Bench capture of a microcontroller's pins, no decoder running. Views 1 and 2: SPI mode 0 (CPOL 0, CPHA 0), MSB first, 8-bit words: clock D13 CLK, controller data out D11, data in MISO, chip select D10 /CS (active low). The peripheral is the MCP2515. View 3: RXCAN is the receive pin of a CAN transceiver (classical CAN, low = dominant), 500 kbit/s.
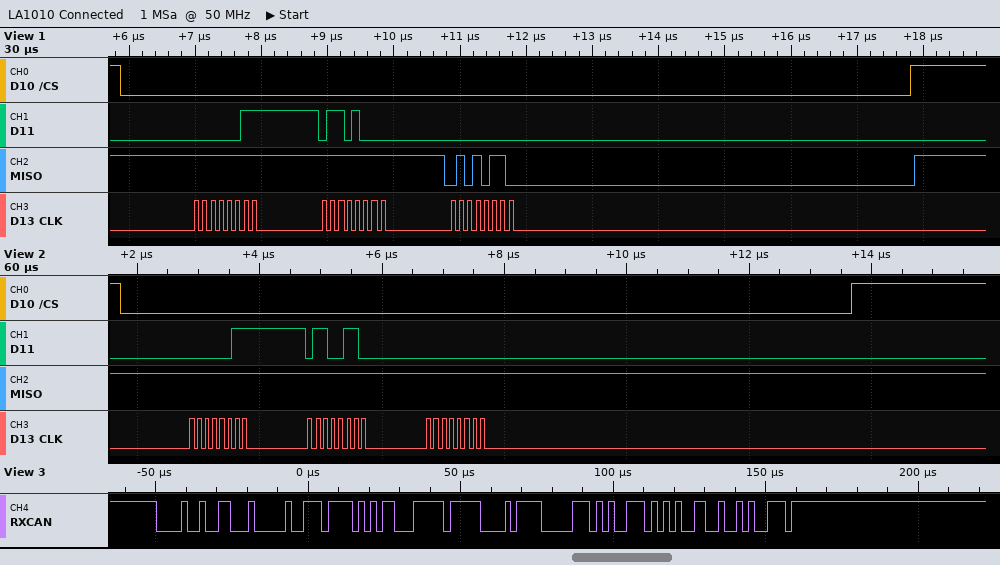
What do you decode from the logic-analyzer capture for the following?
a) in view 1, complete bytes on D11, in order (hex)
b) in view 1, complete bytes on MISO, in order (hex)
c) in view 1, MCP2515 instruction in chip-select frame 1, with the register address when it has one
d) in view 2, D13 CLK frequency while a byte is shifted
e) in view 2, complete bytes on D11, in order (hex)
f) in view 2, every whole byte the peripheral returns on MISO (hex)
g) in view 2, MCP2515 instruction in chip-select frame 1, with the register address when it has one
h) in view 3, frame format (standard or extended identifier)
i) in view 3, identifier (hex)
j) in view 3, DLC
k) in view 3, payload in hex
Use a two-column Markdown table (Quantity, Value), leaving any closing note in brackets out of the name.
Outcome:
| Quantity | Value |
|---|---|
| in view 1, complete bytes on D11, in order | 0x03 0x68 0x00 |
| in view 1, complete bytes on MISO, in order | 0xFF 0xFF 0x56 |
| in view 1, MCP2515 instruction in chip-select frame 1, with the register address when it has one | READ 0x68 |
| in view 2, D13 CLK frequency while a byte is shifted | 8 MHz |
| in view 2, complete bytes on D11, in order | 0x03 0x66 0x00 |
| in view 2, every whole byte the peripheral returns on MISO | 0xFF 0xFF 0xFF |
| in view 2, MCP2515 instruction in chip-select frame 1, with the register address when it has one | READ 0x66 |
| in view 3, frame format | standard |
| in view 3, identifier | 0x093 |
| in view 3, DLC | 8 |
| in view 3, payload in hex | 0E F5 63 FF 17 83 53 AA |
